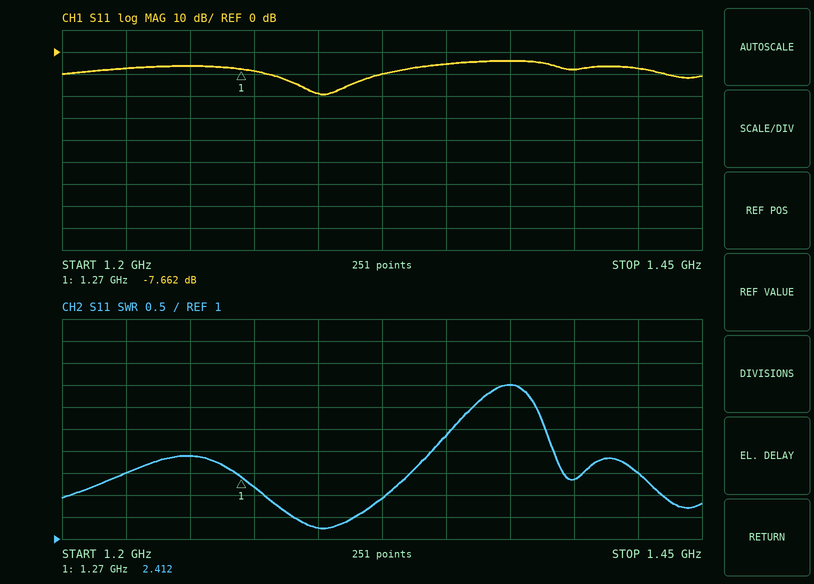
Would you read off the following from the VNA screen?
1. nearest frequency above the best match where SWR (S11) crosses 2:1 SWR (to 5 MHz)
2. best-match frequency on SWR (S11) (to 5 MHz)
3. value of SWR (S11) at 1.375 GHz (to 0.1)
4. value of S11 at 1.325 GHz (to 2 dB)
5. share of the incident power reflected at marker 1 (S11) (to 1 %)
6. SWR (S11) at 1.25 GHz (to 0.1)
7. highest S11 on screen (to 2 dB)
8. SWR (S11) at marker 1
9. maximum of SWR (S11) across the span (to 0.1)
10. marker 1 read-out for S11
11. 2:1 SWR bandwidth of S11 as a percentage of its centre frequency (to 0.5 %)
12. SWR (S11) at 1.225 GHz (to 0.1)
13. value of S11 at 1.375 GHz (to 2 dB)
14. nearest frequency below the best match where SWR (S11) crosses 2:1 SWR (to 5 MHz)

1.325 GHz
1.300 GHz
4.5
-10 dB
17 %
2.9
-4 dB
2.412
4.5
-7.662 dB
3.5 %
2.5
-4 dB
1.280 GHz
